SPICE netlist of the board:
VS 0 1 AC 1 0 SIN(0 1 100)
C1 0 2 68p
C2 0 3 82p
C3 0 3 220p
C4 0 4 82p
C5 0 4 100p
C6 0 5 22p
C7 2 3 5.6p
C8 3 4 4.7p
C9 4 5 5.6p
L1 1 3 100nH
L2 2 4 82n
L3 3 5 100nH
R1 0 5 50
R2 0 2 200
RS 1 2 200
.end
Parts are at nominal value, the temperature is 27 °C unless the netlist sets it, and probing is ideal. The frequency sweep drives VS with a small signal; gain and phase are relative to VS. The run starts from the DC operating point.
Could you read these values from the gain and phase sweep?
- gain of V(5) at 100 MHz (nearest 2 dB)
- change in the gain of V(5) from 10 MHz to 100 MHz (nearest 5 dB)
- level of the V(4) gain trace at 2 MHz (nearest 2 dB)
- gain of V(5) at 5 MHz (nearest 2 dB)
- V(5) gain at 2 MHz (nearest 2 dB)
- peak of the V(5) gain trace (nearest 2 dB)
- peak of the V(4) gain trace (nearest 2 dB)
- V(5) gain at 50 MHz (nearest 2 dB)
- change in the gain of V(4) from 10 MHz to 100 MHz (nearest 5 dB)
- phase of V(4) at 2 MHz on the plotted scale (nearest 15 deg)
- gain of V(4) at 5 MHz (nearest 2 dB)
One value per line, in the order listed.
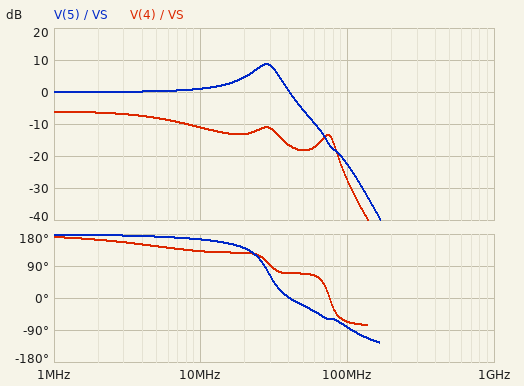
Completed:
-22 dB
-25 dB
-6 dB
0 dB
0 dB
8 dB
-6 dB
-6 dB
-15 dB
165 deg
-8 dB
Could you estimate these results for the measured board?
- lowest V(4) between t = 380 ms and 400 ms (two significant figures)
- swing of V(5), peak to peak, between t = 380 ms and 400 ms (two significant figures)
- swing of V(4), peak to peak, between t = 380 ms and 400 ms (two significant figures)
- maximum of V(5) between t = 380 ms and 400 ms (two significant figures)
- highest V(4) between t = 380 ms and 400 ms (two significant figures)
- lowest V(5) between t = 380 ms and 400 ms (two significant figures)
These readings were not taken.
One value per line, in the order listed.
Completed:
-500 mV
2.0 V
1.0 V
1.0 V
500 mV
-1.0 V
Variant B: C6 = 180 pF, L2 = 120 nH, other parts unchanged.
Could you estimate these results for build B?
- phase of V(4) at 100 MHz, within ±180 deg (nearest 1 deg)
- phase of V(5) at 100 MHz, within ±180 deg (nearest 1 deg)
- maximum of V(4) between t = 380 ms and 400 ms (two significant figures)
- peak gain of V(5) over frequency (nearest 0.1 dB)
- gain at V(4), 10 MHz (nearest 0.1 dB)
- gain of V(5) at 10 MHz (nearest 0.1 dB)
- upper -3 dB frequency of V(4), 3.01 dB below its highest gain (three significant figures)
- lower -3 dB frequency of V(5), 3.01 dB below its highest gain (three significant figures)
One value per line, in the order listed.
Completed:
-70 deg
-164 deg
500 mV
8.3 dB
-10.9 dB
2.2 dB
6.54 MHz
15.1 MHz
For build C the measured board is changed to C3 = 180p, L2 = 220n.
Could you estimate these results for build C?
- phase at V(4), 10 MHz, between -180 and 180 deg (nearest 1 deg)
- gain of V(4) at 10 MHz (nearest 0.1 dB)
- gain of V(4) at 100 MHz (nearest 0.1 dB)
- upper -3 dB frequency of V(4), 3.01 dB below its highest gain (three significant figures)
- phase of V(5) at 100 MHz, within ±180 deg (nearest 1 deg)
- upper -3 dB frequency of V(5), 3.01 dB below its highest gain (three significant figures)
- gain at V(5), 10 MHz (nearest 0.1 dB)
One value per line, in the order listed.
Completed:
129 deg
-10.8 dB
-38.9 dB
6.74 MHz
-86 deg
36.2 MHz
0.9 dB
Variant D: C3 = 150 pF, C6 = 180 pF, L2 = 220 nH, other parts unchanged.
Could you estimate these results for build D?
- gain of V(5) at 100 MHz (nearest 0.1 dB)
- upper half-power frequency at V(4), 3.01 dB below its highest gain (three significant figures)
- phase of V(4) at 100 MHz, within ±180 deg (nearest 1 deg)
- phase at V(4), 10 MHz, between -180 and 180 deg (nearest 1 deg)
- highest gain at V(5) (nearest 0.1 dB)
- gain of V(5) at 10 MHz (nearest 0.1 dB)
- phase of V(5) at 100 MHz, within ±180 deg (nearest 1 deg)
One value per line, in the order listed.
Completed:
-33.7 dB
6.77 MHz
-62 deg
130 deg
7.5 dB
1.9 dB
-166 deg
